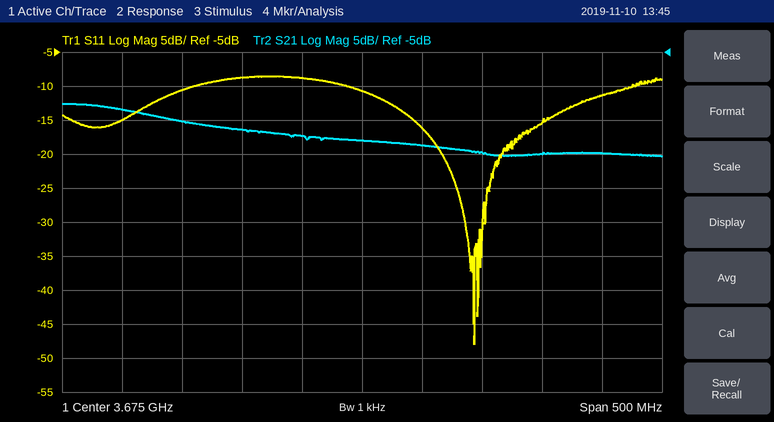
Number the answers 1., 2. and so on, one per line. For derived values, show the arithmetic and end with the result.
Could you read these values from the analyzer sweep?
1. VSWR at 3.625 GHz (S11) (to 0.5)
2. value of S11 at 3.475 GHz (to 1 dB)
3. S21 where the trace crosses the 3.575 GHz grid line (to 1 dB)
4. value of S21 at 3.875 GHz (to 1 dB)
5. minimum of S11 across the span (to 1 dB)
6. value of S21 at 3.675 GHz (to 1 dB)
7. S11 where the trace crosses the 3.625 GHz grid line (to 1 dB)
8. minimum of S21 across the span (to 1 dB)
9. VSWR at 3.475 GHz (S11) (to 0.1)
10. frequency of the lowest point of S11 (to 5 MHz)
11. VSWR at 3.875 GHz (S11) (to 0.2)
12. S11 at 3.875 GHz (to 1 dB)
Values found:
1. |Γ| = 10^(-9/20) = 0.3548; VSWR = (1 + 0.3548)/(1 − 0.3548) ≈ 2.10, so 2.0 to the nearest 0.5
2. -15 dB
3. -16 dB
4. -20 dB
5. -48 dB
6. -18 dB
7. -9 dB
8. -20 dB
9. |Γ| = 10^(-15/20) = 0.1778; VSWR = (1 + 0.1778)/(1 − 0.1778) ≈ 1.4
10. 3.770 GHz
11. |Γ| = 10^(-11/20) = 0.2818; VSWR = (1 + 0.2818)/(1 − 0.2818) ≈ 1.8
12. -11 dB
